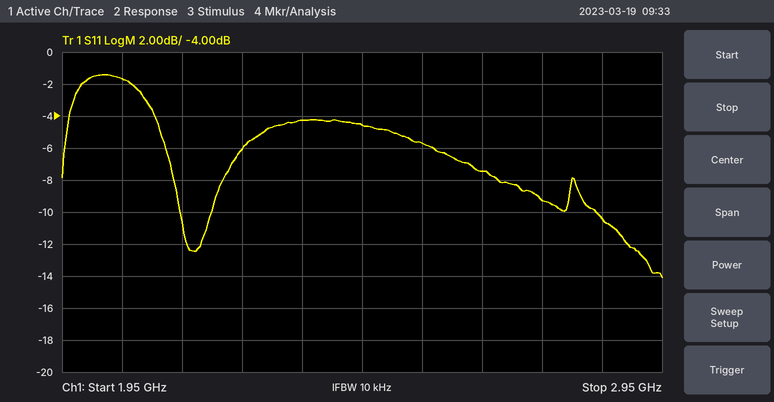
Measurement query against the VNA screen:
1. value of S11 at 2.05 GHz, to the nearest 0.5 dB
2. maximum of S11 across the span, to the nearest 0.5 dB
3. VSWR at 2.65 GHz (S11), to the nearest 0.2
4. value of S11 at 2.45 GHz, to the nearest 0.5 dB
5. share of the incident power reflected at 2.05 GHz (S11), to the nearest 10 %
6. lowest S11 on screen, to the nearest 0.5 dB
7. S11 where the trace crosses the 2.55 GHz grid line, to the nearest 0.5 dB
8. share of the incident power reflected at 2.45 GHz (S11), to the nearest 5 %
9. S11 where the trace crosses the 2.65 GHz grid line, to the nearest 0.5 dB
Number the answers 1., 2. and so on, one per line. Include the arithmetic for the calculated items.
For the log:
1. -1.5 dB
2. -1.5 dB
3. |Γ| = 10^(-7.5/20) = 0.4217; VSWR = (1 + 0.4217)/(1 − 0.4217) ≈ 2.46, so 2.4 to the nearest 0.2
4. -4.5 dB
5. 10^(-1.5/10) ≈ 70.8 %, so 70 % to the nearest 10 %
6. -14.0 dB
7. -5.5 dB
8. 10^(-4.5/10) ≈ 35 %
9. -7.5 dB
